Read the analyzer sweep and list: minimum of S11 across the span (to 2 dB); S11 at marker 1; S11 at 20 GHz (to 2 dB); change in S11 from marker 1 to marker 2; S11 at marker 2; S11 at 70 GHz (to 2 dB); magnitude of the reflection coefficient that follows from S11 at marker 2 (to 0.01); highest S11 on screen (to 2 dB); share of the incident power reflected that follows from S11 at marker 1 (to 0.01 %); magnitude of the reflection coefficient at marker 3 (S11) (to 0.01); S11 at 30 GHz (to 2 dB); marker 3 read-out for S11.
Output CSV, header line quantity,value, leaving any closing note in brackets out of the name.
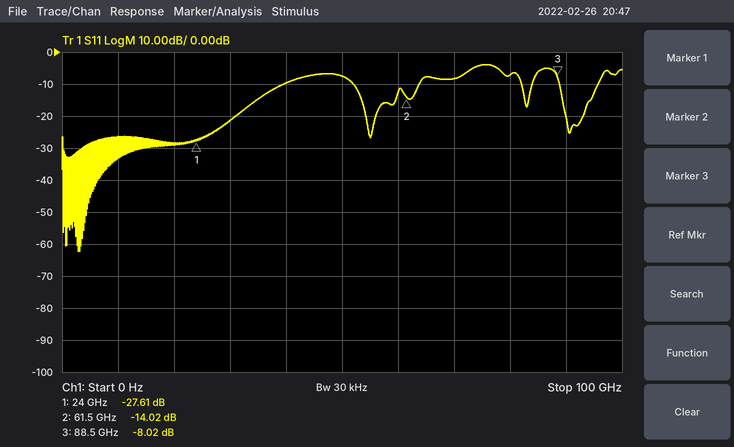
quantity,value
minimum of S11 across the span,-62 dB
S11 at marker 1,-27.61 dB
S11 at 20 GHz,-28 dB
change in S11 from marker 1 to marker 2,13.59 dB
S11 at marker 2,-14.02 dB
S11 at 70 GHz,-8 dB
magnitude of the reflection coefficient that follows from S11 at marker 2,0.20
highest S11 on screen,-4 dB
share of the incident power reflected that follows from S11 at marker 1,0.17 %
magnitude of the reflection coefficient at marker 3 (S11),0.40
S11 at 30 GHz,-22 dB
marker 3 read-out for S11,-8.02 dB
